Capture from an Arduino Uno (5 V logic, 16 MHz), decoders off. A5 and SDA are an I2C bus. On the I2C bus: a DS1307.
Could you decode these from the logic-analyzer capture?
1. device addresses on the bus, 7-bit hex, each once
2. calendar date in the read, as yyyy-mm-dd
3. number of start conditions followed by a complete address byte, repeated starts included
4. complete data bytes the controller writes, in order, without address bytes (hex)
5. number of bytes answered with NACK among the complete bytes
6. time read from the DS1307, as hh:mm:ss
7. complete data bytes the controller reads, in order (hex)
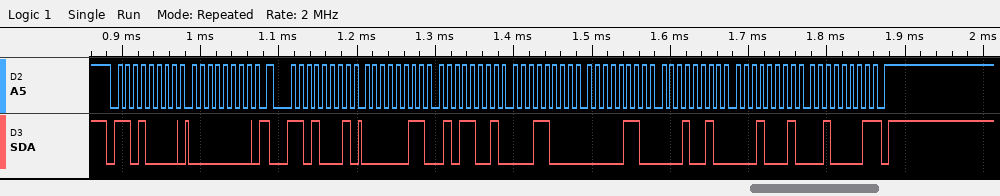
0x68
2021-11-12
2
00
1
18:59:03
03 59 18 06 12 11 21
